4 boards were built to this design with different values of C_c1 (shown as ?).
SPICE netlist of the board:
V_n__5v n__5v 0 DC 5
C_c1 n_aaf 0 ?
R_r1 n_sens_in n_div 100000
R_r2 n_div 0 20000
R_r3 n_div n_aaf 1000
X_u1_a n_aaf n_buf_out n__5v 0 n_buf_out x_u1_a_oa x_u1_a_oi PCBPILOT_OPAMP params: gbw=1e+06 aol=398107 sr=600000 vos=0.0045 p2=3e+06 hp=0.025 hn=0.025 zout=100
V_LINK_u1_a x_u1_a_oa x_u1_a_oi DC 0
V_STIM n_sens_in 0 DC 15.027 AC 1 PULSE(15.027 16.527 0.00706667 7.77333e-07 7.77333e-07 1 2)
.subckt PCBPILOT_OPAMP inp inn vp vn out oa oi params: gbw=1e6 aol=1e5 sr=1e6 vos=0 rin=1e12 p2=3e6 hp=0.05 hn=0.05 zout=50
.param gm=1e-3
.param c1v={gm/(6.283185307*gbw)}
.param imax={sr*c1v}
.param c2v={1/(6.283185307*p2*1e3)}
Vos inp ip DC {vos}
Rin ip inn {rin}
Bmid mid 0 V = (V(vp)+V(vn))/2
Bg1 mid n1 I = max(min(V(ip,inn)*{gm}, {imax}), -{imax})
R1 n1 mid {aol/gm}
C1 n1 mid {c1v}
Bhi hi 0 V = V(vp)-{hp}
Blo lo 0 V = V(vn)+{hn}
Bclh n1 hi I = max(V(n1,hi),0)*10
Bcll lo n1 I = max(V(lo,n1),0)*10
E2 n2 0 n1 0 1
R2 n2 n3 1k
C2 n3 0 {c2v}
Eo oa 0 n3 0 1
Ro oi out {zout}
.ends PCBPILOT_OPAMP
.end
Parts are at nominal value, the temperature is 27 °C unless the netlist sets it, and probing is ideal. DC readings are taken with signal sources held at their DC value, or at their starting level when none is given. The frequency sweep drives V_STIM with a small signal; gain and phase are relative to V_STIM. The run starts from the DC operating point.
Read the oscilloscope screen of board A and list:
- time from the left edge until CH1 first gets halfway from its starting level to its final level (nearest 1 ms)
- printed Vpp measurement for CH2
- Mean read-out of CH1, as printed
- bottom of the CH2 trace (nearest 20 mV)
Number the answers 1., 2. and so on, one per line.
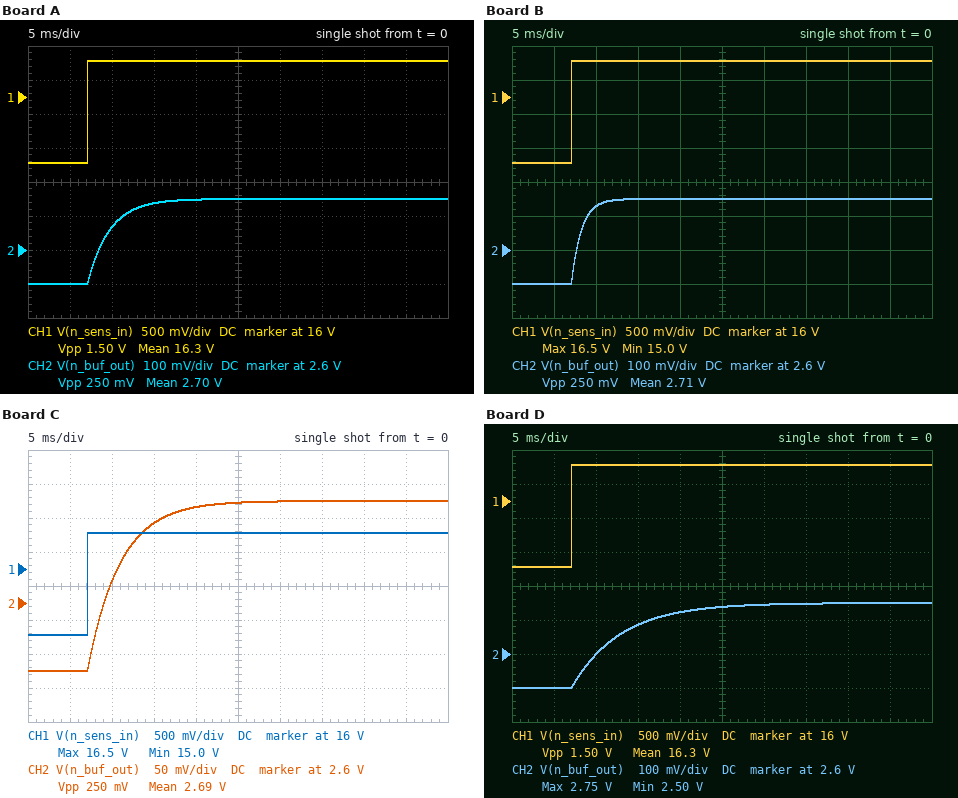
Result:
1. 7 ms
2. 250 mV
3. 16.3 V
4. 2.50 V
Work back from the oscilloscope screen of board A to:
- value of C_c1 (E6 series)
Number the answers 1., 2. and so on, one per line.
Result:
1. 150 nF
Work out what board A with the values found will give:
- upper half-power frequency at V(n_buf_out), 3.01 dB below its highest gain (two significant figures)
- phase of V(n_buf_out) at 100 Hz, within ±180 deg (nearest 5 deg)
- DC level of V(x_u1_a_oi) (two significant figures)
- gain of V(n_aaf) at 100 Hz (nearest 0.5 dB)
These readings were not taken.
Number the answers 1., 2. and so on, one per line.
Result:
1. 60 Hz
2. -60 deg
3. 2.5 V
4. -21.5 dB
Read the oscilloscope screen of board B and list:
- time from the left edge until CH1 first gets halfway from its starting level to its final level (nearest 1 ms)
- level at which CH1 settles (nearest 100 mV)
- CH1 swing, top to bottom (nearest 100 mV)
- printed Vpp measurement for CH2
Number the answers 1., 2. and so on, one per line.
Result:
1. 7 ms
2. 16.5 V
3. 1.5 V
4. 250 mV
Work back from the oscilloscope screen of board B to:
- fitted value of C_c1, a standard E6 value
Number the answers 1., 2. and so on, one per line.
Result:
1. 68 nF
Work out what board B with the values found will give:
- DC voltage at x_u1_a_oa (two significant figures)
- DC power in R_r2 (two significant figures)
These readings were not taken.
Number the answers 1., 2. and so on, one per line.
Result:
1. 2.5 V
2. 310 µW
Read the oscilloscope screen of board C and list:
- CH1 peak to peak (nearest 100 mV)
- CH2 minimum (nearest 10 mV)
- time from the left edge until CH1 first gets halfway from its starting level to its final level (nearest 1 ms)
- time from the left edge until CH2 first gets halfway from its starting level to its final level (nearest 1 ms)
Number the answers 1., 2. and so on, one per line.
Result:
1. 1.5 V
2. 2.50 V
3. 7 ms
4. 10 ms
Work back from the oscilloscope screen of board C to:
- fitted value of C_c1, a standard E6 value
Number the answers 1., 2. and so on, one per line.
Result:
1. 220 nF
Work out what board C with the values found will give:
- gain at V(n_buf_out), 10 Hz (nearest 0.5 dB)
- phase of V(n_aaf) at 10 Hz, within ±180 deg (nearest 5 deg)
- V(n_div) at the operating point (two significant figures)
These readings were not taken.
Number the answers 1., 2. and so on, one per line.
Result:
1. -16.0 dB
2. -15 deg
3. 2.5 V
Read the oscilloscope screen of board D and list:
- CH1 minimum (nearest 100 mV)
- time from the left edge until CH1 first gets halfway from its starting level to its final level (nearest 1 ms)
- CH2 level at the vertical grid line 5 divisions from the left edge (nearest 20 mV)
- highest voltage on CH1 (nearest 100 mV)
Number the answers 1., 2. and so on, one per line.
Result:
1. 15.0 V
2. 7 ms
3. 2.74 V
4. 16.5 V
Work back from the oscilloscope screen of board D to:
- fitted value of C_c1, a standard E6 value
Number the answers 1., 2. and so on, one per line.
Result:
1. 330 nF
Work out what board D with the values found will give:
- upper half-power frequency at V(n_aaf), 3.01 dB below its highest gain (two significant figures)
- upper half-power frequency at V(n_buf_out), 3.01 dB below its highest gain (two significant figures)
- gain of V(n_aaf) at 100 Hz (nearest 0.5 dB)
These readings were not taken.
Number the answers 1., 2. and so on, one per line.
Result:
1. 27 Hz
2. 27 Hz
3. -27.0 dB
